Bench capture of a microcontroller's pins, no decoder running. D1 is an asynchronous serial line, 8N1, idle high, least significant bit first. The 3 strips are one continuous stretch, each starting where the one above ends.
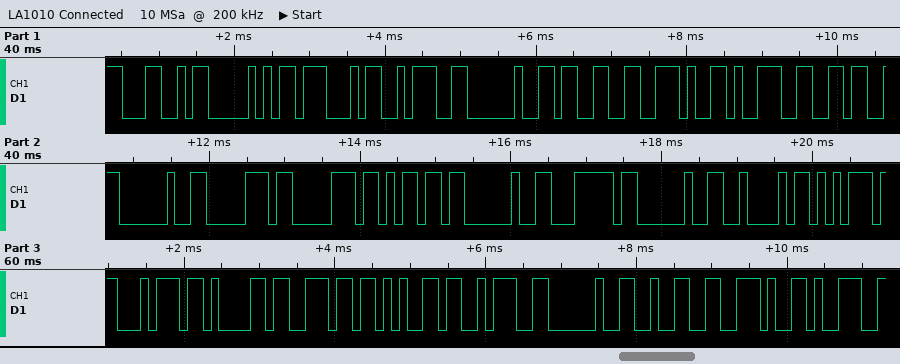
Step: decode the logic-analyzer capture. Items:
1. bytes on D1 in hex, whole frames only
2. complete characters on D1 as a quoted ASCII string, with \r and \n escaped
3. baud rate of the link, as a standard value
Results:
0x4C 0x50 0x47 0x3A 0x20 0x33 0x2E 0x39 0x36 0x20 0x70 0x70 0x6D 0x20 0x7C 0x20 0x42 0x75 0x74 0x61 0x6E 0x65 0x3A 0x20 0x32 0x2E 0x39
"LPG: 3.96 ppm | Butane: 2.9"
9600 baud
